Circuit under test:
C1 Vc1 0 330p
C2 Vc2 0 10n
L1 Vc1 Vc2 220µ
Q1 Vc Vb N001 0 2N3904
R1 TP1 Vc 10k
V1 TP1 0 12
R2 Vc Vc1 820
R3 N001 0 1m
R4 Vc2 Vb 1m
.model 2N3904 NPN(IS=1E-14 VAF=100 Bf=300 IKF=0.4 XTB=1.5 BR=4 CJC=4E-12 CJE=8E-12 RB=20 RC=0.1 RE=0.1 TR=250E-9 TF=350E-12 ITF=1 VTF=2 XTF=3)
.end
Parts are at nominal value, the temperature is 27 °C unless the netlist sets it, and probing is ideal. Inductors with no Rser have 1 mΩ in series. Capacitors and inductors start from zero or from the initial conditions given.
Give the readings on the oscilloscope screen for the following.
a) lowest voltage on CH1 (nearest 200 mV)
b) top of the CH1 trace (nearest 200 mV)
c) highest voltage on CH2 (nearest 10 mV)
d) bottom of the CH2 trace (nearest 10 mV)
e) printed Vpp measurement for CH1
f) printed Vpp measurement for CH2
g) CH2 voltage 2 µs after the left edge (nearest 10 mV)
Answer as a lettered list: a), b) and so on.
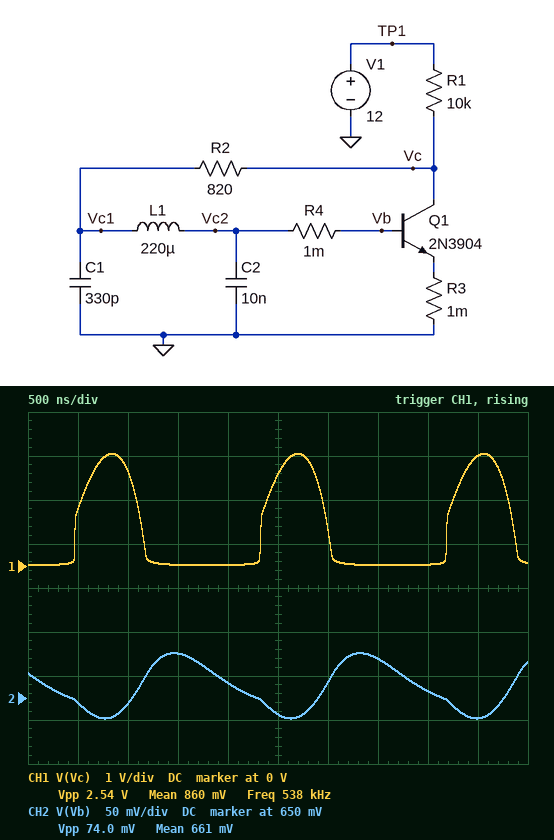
a) 0 V
b) 2.6 V
c) 700 mV
d) 630 mV
e) 2.54 V
f) 74.0 mV
g) 670 mV
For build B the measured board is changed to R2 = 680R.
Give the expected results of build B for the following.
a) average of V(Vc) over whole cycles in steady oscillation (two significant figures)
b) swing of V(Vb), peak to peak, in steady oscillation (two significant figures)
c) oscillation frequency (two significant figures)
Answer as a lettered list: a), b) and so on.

a) 760 mV
b) 76 mV
c) 530 kHz
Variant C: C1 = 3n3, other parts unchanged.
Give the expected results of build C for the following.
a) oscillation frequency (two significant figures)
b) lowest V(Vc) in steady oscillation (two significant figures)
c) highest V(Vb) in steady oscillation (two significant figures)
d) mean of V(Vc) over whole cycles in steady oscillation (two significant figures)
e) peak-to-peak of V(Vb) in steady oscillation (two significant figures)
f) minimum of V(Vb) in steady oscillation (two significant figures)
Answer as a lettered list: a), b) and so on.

a) 210 kHz
b) -17 mV
c) 800 mV
d) 1.1 V
e) 580 mV
f) 220 mV
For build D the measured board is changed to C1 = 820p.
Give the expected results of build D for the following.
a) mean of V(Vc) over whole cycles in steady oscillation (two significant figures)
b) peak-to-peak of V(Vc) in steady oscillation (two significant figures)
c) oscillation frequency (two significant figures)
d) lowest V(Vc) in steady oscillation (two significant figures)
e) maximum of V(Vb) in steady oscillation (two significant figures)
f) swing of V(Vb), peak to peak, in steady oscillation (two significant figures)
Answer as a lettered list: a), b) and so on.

a) 950 mV
b) 2.9 V
c) 370 kHz
d) 4.6 mV
e) 750 mV
f) 180 mV
